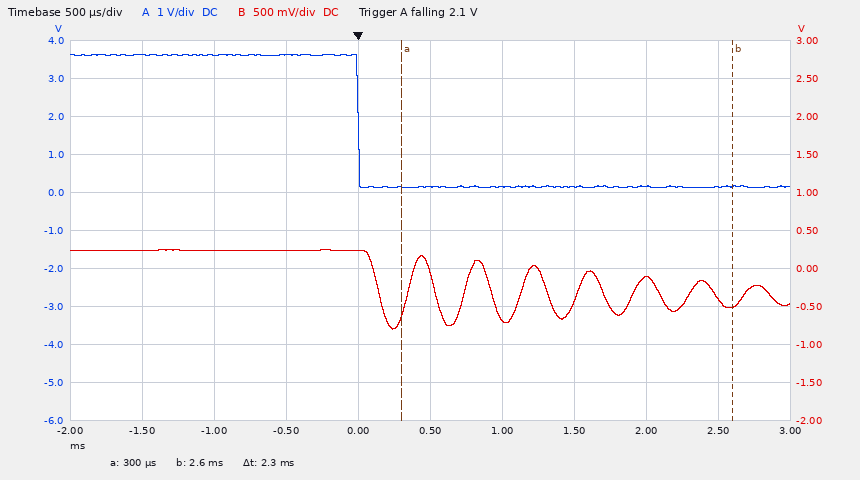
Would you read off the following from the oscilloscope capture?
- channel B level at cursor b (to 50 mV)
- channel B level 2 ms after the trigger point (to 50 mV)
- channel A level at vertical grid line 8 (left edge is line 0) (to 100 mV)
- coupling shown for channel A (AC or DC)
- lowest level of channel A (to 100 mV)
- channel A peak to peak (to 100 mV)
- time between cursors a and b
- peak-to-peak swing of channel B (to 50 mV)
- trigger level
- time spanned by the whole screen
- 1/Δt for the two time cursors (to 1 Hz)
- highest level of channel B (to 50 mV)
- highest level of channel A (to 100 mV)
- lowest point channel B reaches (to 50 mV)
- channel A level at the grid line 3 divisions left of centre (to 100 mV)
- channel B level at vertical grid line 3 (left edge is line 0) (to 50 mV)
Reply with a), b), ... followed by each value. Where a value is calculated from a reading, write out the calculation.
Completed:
a) -500 mV
b) -100 mV
c) 200 mV
d) DC
e) 100 mV
f) 3.6 V − (100 mV) = 3.5 V
g) 2.3 ms
h) 250 mV − (-800 mV) = 1.05 V
i) 2.1 V
j) 5 ms
k) 1 / 2.3 ms ≈ 435 Hz
l) 250 mV
m) 3.6 V
n) -800 mV
o) 3.6 V
p) 250 mV
